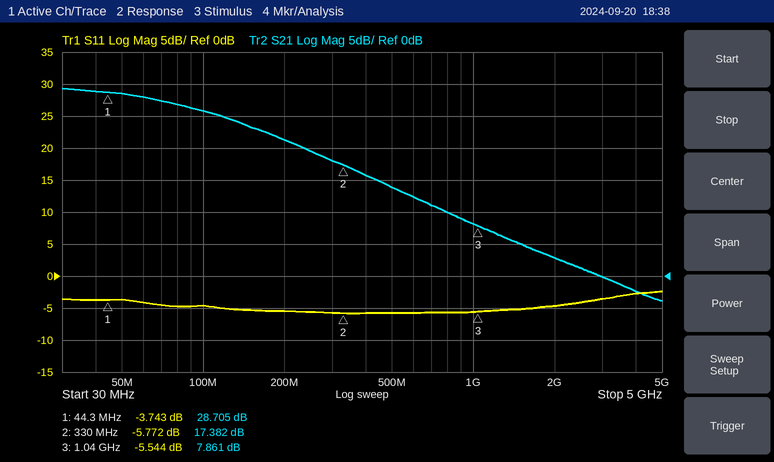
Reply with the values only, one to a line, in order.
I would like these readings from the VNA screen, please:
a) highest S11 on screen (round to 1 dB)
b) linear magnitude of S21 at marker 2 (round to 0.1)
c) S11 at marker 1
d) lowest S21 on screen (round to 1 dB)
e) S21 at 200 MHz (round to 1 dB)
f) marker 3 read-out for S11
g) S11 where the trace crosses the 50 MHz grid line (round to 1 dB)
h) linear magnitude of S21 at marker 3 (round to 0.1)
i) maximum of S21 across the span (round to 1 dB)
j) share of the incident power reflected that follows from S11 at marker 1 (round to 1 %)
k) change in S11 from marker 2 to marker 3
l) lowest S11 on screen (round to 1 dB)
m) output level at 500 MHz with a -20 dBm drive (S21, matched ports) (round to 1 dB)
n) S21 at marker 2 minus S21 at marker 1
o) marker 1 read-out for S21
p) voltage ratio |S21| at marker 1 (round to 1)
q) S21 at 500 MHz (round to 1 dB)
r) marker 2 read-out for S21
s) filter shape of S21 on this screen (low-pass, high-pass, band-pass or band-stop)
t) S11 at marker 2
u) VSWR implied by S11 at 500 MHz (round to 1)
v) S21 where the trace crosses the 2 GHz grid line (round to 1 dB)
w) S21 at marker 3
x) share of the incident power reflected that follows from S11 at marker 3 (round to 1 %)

-2 dB
7.4
-3.743 dB
-4 dB
21 dB
-5.544 dB
-4 dB
2.5
29 dB
42 %
0.228 dB
-6 dB
-6 dBm
-11.323 dB
28.705 dB
27
14 dB
17.382 dB
low-pass
-5.772 dB
3
3 dB
7.861 dB
28 %
